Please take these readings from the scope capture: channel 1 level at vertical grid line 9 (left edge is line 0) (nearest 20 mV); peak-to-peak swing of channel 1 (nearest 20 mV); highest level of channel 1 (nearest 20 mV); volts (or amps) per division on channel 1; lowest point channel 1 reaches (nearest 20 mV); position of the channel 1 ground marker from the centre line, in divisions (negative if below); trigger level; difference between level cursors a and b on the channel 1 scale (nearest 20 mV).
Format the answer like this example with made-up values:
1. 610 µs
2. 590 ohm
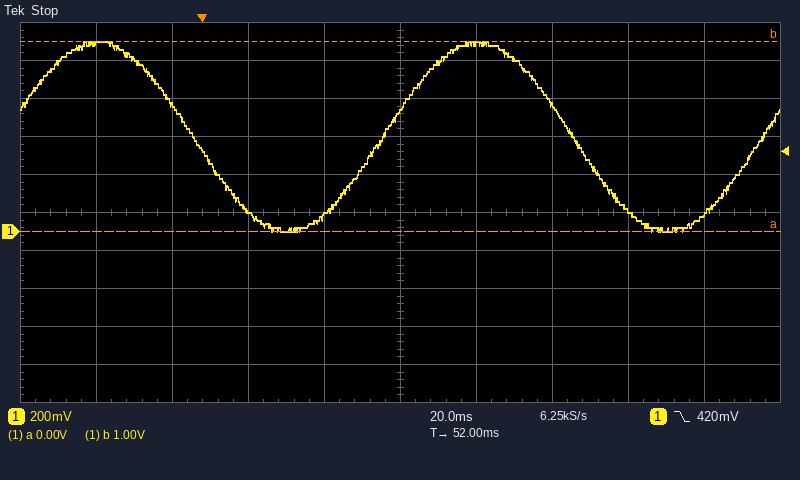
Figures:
1. 100 mV
2. 1.00 V
3. 1.00 V
4. 200 mV
5. 0 mV
6. -0.5 div
7. 420 mV
8. 1.00 V
